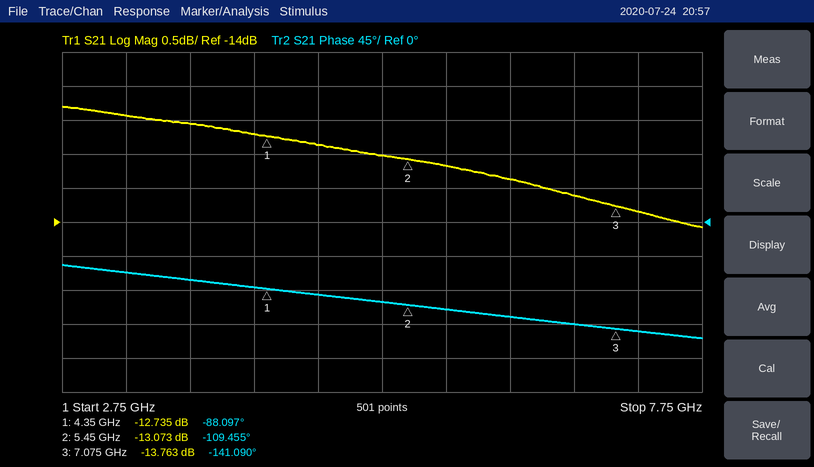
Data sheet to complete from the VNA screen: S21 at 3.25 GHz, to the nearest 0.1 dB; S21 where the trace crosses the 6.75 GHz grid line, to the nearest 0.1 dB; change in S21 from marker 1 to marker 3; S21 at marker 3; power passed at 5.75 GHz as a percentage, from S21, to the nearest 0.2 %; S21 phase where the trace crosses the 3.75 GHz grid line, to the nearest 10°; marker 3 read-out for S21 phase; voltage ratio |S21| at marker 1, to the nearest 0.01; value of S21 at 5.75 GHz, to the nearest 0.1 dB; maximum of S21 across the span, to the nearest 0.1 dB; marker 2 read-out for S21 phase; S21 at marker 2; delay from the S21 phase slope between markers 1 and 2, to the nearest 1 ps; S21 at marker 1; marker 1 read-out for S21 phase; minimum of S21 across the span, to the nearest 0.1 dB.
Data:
-12.4 dB
-13.6 dB
-1.028 dB
-13.763 dB
4.8 %
-80°
-141.090°
0.23
-13.2 dB
-12.3 dB
-109.455°
-13.073 dB
54 ps
-12.735 dB
-88.097°
-14.1 dB
